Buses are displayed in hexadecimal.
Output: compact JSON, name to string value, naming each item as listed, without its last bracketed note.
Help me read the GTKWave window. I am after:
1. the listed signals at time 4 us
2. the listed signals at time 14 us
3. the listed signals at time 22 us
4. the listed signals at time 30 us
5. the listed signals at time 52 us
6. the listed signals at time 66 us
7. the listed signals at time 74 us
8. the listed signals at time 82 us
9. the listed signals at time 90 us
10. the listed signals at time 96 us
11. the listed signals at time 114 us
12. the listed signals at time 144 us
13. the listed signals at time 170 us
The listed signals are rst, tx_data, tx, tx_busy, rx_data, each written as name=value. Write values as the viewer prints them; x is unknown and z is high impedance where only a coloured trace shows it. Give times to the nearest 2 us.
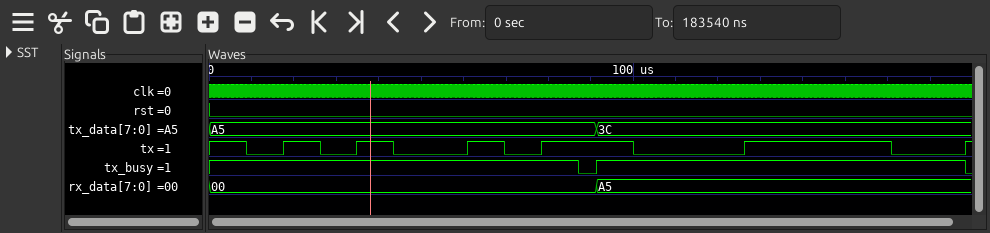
{"the listed signals at time 4 us": "rst=0, tx_data=A5, tx=1, tx_busy=1, rx_data=00", "the listed signals at time 14 us": "rst=0, tx_data=A5, tx=0, tx_busy=1, rx_data=00", "the listed signals at time 22 us": "rst=0, tx_data=A5, tx=1, tx_busy=1, rx_data=00", "the listed signals at time 30 us": "rst=0, tx_data=A5, tx=0, tx_busy=1, rx_data=00", "the listed signals at time 52 us": "rst=0, tx_data=A5, tx=0, tx_busy=1, rx_data=00", "the listed signals at time 66 us": "rst=0, tx_data=A5, tx=1, tx_busy=1, rx_data=00", "the listed signals at time 74 us": "rst=0, tx_data=A5, tx=0, tx_busy=1, rx_data=00", "the listed signals at time 82 us": "rst=0, tx_data=A5, tx=1, tx_busy=1, rx_data=00", "the listed signals at time 90 us": "rst=0, tx_data=A5, tx=1, tx_busy=0, rx_data=00", "the listed signals at time 96 us": "rst=0, tx_data=3C, tx=1, tx_busy=1, rx_data=A5", "the listed signals at time 114 us": "rst=0, tx_data=3C, tx=0, tx_busy=1, rx_data=A5", "the listed signals at time 144 us": "rst=0, tx_data=3C, tx=1, tx_busy=1, rx_data=A5", "the listed signals at time 170 us": "rst=0, tx_data=3C, tx=0, tx_busy=1, rx_data=A5"}
